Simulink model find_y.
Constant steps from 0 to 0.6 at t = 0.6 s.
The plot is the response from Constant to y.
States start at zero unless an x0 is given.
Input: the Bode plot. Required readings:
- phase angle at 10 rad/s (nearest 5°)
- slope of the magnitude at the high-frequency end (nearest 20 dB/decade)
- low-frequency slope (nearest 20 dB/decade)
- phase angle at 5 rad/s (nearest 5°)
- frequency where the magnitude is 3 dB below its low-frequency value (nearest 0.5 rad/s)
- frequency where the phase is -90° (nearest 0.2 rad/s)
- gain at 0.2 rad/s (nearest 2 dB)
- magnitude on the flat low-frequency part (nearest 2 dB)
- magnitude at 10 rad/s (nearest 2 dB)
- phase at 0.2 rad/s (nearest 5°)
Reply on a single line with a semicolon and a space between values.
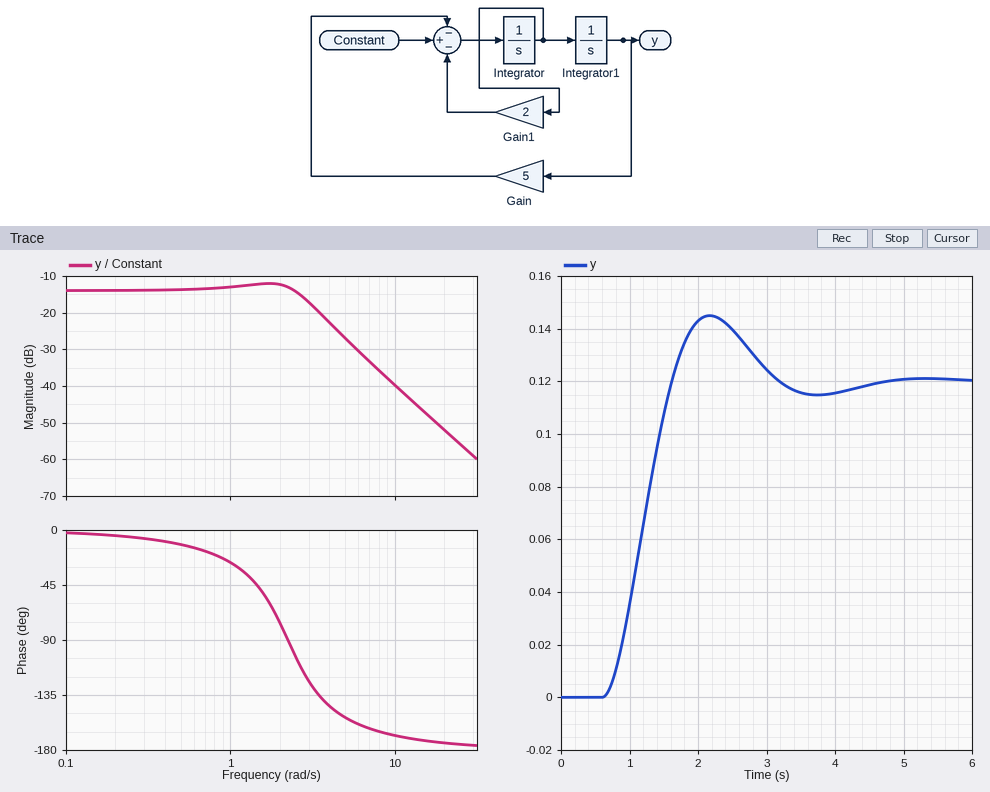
-170°; -40 dB/decade; 0 dB/decade; -155°; 3.0 rad/s; 2.2 rad/s; -14 dB; -14 dB; -40 dB; -5°
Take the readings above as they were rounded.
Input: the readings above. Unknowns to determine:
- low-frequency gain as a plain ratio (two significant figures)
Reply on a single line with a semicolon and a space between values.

0.20
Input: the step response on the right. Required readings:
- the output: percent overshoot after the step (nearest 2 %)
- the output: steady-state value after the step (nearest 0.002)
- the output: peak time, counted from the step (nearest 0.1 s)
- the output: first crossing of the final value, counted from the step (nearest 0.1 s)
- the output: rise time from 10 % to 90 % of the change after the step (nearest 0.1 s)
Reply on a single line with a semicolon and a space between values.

20 %; 0.120; 1.6 s; 1.0 s; 0.7 s
